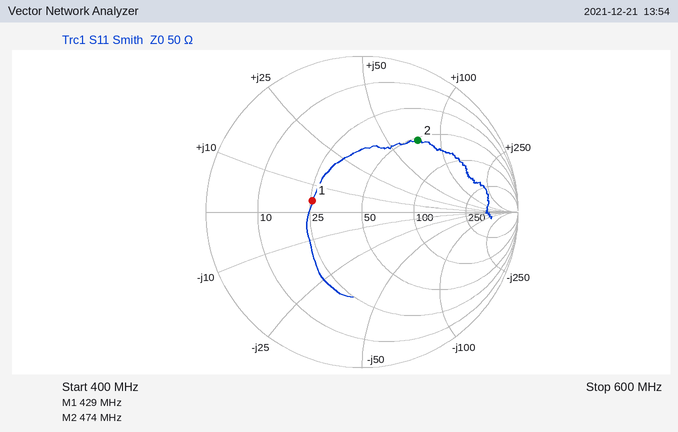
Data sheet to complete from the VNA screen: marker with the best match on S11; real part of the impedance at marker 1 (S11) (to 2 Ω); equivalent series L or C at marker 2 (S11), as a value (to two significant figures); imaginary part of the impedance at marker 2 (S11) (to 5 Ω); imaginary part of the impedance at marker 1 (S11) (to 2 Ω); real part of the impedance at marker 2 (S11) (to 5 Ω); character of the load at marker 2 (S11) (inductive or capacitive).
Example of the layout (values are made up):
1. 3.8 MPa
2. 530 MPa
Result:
1. marker 1
2. 26 Ω
3. 25 nH
4. +75 Ω
5. +4 Ω
6. 55 Ω
7. inductive
